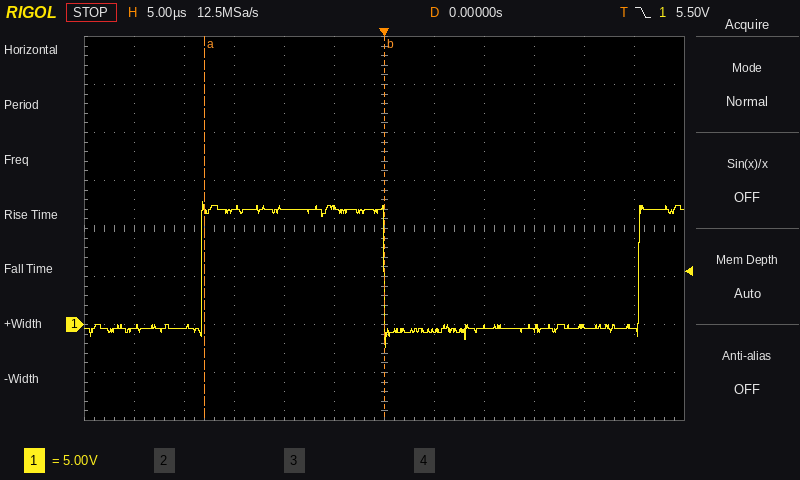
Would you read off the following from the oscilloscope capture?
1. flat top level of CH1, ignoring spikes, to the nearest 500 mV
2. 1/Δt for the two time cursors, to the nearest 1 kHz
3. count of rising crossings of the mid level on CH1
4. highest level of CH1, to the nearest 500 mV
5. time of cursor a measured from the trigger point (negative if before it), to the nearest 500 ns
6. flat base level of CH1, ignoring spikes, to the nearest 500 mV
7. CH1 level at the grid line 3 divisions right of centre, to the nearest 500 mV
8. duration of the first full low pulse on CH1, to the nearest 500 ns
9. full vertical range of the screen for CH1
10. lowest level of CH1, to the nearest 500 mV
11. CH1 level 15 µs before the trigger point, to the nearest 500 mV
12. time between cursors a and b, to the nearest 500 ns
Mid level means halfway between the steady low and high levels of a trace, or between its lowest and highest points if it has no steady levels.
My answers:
12.0 V
56 kHz
2
13.0 V
-18.0 µs
-500 mV
-500 mV
25.5 µs
40 V
-2.5 V
12.0 V
18.0 µs
